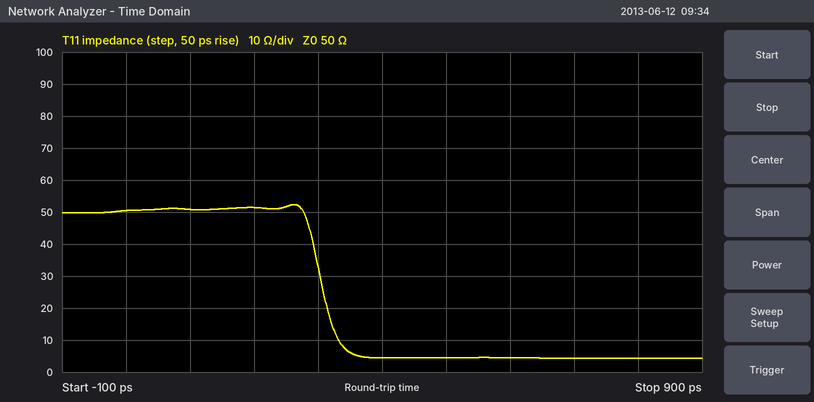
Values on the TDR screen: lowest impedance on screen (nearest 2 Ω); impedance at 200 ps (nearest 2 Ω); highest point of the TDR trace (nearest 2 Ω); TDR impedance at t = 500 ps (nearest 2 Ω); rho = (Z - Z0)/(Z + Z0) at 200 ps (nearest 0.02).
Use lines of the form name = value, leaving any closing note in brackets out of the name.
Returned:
lowest impedance on screen = 4 Ω
impedance at 200 ps = 52 Ω
highest point of the TDR trace = 52 Ω
TDR impedance at t = 500 ps = 4 Ω
rho = (Z - Z0)/(Z + Z0) at 200 ps = +0.02
